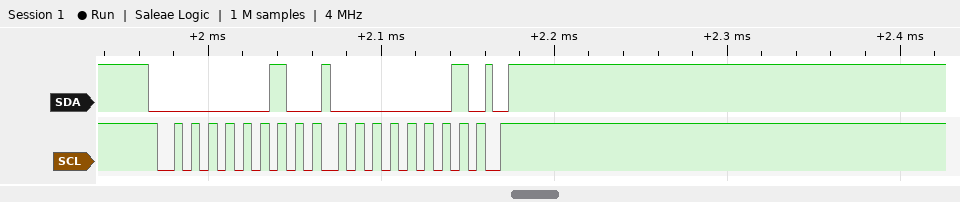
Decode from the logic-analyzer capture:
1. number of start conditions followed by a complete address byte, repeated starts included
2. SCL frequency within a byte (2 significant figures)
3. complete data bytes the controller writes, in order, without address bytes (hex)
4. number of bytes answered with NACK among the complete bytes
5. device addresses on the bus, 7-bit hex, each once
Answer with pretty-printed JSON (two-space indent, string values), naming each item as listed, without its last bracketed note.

{
  "number of start conditions followed by a complete address byte, repeated starts included": "1",
  "SCL frequency within a byte": "100 kHz",
  "complete data bytes the controller writes, in order, without address bytes": "01",
  "number of bytes answered with NACK among the complete bytes": "0",
  "device addresses on the bus, 7-bit hex, each once": "0x01"
}
